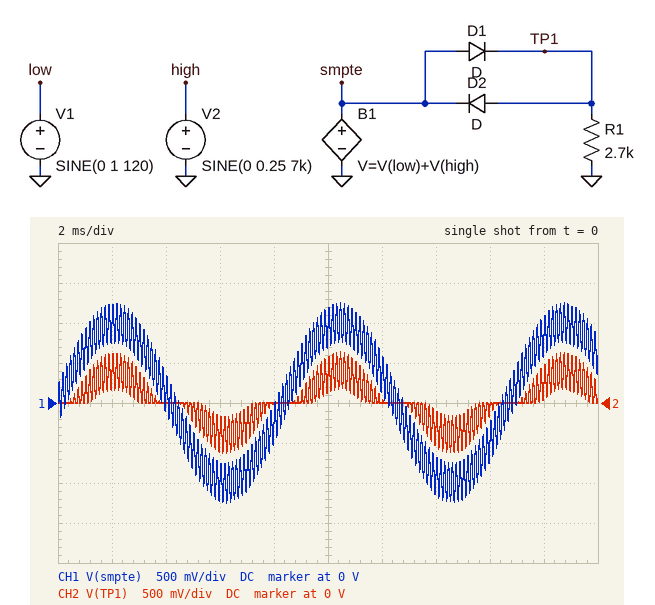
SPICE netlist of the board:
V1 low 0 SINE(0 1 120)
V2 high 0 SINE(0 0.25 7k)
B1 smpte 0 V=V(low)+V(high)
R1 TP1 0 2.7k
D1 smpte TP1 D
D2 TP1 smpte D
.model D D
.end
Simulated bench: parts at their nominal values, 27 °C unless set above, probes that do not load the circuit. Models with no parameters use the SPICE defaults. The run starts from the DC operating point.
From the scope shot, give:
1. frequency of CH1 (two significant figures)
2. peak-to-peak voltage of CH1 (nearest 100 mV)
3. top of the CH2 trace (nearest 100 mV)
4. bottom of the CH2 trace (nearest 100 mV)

120 Hz
2.5 V
600 mV
-600 mV
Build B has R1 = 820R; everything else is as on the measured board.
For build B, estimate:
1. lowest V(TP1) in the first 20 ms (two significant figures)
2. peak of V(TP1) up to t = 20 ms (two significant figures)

-600 mV
600 mV
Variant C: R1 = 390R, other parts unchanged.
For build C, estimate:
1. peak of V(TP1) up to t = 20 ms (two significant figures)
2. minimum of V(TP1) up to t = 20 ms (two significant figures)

580 mV
-580 mV
